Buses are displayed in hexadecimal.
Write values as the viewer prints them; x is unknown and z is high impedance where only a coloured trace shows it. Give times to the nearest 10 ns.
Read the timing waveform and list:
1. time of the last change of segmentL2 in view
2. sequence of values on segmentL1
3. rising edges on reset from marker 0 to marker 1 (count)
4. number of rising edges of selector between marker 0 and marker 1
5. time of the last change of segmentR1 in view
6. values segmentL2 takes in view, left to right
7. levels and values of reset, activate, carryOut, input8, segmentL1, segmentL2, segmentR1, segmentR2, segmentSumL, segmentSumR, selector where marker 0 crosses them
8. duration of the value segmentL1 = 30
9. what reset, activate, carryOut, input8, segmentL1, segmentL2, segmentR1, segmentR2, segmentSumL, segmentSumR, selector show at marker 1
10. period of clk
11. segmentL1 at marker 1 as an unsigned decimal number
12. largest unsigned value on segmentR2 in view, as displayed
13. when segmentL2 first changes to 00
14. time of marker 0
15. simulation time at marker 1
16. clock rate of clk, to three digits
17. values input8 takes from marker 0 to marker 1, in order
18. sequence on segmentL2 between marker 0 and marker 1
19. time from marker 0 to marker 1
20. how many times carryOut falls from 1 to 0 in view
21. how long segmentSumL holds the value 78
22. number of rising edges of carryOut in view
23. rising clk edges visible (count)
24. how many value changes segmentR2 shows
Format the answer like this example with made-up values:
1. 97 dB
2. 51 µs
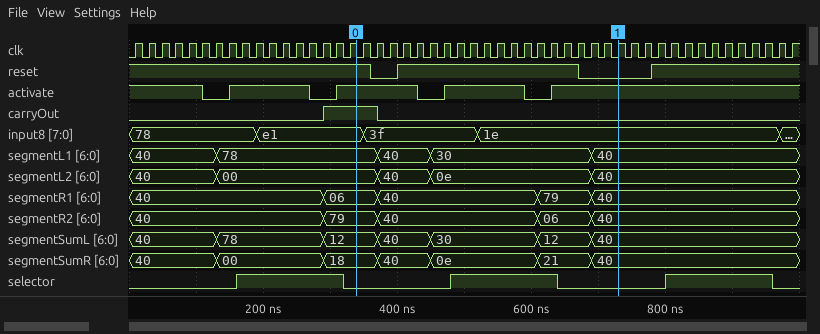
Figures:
1. 690 ns
2. 40, 78, 40, 30, 40
3. 1
4. 1
5. 690 ns
6. 40, 00, 40, 0e, 40
7. reset=1, activate=1, carryOut=1, input8=e1, segmentL1=78, segmentL2=00, segmentR1=06, segmentR2=79, segmentSumL=12, segmentSumR=18, selector=0
8. 240 ns
9. reset=0, activate=1, carryOut=0, input8=1e, segmentL1=40, segmentL2=40, segmentR1=40, segmentR2=40, segmentSumL=40, segmentSumR=40, selector=0
10. 20 ns
11. 64
12. 79
13. 130 ns
14. 340 ns
15. 730 ns
16. 50.0 MHz
17. e1, 3f, 1e
18. 00, 40, 0e, 40
19. 390 ns
20. 1
21. 160 ns
22. 1
23. 50
24. 4
